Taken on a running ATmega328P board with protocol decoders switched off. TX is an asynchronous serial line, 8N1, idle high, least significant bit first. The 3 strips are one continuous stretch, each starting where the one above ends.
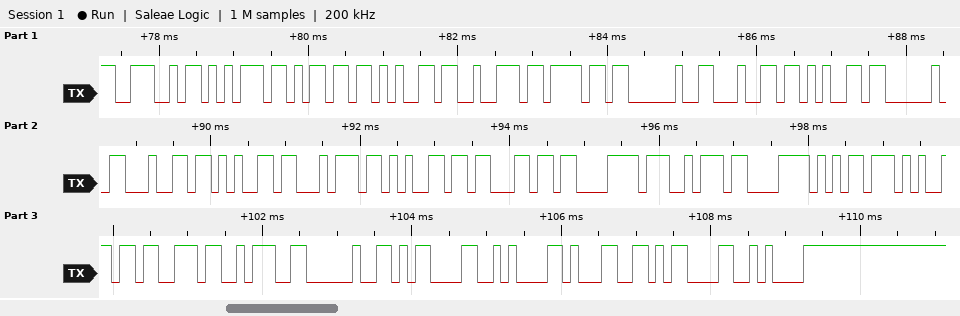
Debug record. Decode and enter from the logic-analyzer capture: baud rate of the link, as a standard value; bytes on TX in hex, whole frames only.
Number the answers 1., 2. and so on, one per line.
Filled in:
1. 9600 baud
2. 0x4E 0x75 0x6D 0x65 0x72 0x6F 0x20 0x64 0x65 0x20 0x64 0x65 0x74 0x65 0x63 0xC3 0xA7 0xC3 0xB5 0x65 0x73 0x3A 0x20 0x0D 0x0A 0x31 0x0D 0x0A
